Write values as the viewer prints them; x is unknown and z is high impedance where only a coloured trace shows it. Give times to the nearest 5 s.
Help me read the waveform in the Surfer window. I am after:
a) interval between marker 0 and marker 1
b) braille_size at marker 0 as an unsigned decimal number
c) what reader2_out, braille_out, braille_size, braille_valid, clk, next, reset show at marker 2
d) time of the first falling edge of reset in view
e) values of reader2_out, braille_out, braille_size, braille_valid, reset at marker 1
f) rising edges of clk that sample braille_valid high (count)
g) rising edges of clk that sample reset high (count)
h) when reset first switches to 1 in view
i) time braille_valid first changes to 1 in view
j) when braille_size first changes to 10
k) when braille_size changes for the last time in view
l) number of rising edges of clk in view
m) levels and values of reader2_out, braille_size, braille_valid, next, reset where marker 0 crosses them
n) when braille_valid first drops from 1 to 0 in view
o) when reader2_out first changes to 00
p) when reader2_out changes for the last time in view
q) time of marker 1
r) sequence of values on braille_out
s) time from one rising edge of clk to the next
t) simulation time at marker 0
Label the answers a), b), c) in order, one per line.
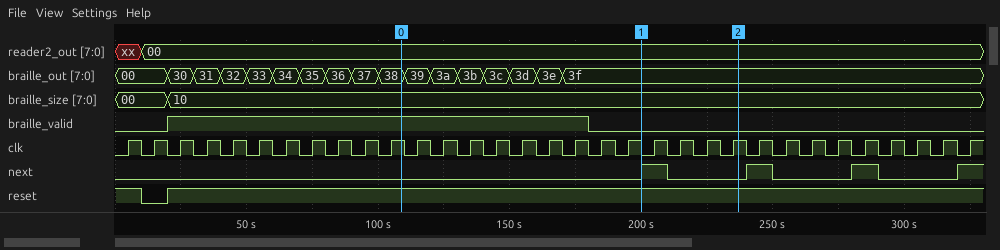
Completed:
a) 90 s
b) 16
c) reader2_out=00, braille_out=3f, braille_size=10, braille_valid=0, clk=1, next=0, reset=1
d) 10 s
e) reader2_out=00, braille_out=3f, braille_size=10, braille_valid=0, reset=1
f) 16
g) 32
h) 20 s
i) 20 s
j) 20 s
k) 20 s
l) 33
m) reader2_out=00, braille_size=10, braille_valid=1, next=0, reset=1
n) 180 s
o) 10 s
p) 10 s
q) 200 s
r) 00, 30, 31, 32, 33, 34, 35, 36, 37, 38, 39, 3a, 3b, 3c, 3d, 3e, 3f
s) 10 s
t) 110 s
